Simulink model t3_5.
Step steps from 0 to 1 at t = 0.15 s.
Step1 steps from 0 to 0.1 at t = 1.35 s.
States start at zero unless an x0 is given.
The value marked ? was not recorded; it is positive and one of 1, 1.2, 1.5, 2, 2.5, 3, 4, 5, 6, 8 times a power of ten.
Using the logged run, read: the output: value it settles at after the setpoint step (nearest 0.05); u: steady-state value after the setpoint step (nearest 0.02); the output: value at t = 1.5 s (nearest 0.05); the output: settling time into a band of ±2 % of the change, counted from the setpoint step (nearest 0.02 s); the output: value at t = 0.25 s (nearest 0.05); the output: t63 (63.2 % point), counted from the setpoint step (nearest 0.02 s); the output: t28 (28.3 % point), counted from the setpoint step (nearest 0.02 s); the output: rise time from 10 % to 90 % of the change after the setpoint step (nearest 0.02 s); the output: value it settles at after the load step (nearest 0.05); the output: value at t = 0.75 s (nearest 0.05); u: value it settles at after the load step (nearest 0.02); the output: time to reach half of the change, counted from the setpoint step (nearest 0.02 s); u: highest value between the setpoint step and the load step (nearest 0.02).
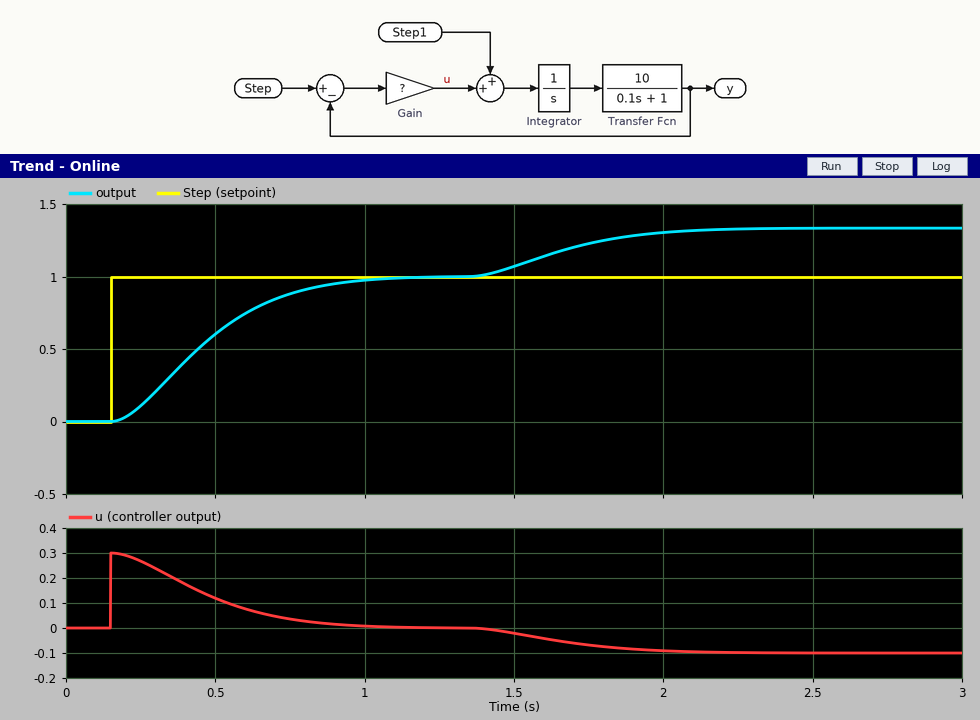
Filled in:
1.00
0.00
1.05
0.88 s
0.10
0.36 s
0.18 s
0.54 s
1.35
0.90
-0.10
0.30 s
0.30
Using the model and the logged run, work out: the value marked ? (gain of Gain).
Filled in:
0.3
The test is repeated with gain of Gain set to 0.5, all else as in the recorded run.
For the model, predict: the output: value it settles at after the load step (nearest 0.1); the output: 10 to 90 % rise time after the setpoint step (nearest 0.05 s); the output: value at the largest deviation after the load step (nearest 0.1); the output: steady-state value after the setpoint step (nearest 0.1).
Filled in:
1.2
0.30 s
1.2
1.0
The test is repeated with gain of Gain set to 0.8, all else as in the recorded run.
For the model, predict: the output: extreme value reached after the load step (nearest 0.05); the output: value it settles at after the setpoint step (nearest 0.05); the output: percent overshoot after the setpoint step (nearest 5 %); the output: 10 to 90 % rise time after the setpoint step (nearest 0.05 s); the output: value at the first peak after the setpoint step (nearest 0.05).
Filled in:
1.15
1.00
10 %
0.20 s
1.10
